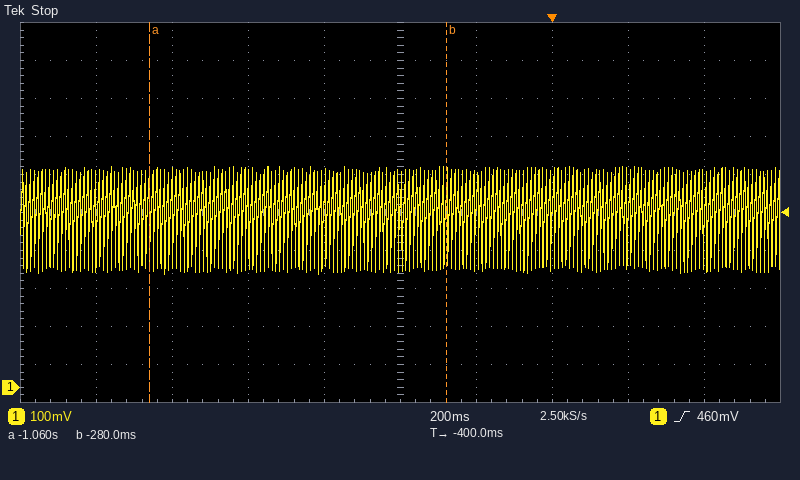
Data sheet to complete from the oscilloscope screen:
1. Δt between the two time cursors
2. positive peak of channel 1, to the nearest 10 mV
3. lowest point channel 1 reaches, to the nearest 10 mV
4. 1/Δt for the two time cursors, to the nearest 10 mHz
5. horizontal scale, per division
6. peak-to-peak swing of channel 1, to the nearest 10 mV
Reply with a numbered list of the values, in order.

1. 780 ms
2. 580 mV
3. 300 mV
4. 1.28 Hz
5. 200 ms
6. 280 mV
